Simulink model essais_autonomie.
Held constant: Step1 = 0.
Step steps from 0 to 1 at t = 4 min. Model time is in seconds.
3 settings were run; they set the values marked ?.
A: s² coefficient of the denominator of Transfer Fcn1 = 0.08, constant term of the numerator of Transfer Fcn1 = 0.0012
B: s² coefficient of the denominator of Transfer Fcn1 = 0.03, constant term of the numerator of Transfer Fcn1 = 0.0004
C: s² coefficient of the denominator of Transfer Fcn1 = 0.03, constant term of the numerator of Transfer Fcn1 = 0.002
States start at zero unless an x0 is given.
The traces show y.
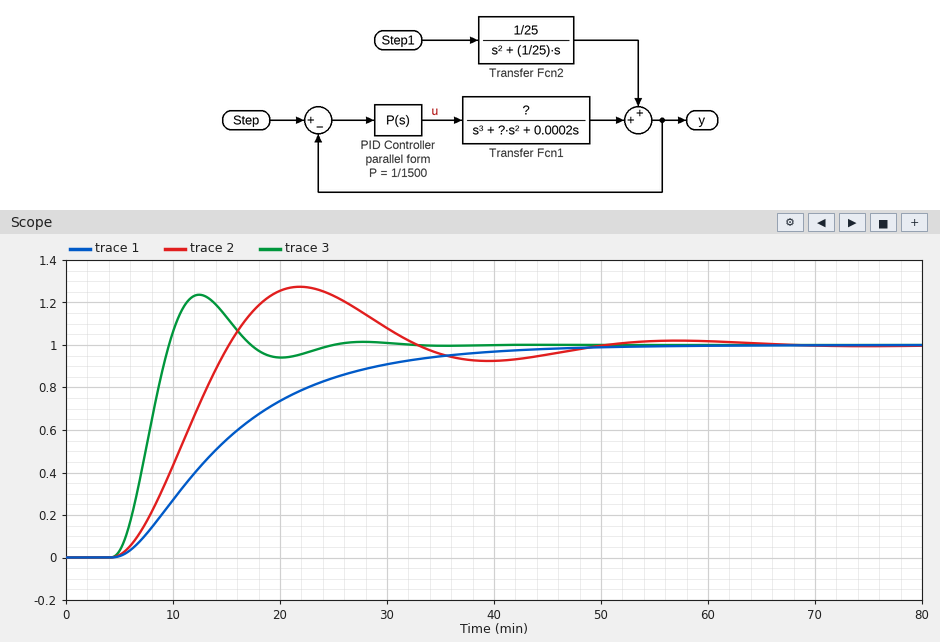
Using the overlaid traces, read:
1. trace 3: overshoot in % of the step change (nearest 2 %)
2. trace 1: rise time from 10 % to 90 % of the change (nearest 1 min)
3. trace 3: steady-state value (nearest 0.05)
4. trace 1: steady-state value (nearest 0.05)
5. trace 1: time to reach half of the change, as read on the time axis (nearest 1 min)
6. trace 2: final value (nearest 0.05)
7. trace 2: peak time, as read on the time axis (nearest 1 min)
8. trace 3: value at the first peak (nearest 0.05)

24 %
22 min
1.00
1.00
14 min
1.00
22 min
1.25
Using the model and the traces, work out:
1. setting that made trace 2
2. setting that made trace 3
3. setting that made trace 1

A
C
B
